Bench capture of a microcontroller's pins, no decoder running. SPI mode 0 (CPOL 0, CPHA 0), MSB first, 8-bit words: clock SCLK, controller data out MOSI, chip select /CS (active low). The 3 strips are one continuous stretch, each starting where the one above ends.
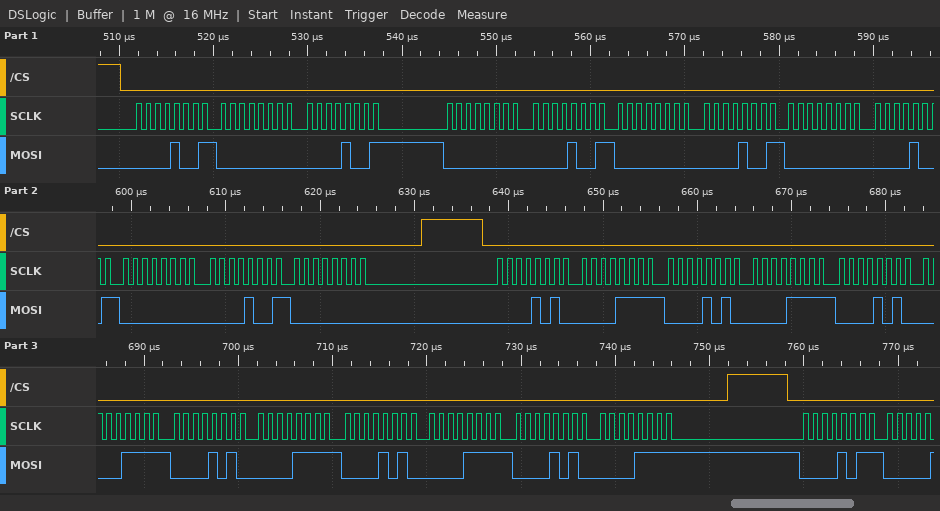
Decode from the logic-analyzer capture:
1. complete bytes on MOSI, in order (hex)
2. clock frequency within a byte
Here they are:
09 00 09 00 09 00 09 00 09 00 09 00 0A 0F 0A 0F 0A 0F 0A 0F 0A 0F 0A 0F 0B
1 MHz
